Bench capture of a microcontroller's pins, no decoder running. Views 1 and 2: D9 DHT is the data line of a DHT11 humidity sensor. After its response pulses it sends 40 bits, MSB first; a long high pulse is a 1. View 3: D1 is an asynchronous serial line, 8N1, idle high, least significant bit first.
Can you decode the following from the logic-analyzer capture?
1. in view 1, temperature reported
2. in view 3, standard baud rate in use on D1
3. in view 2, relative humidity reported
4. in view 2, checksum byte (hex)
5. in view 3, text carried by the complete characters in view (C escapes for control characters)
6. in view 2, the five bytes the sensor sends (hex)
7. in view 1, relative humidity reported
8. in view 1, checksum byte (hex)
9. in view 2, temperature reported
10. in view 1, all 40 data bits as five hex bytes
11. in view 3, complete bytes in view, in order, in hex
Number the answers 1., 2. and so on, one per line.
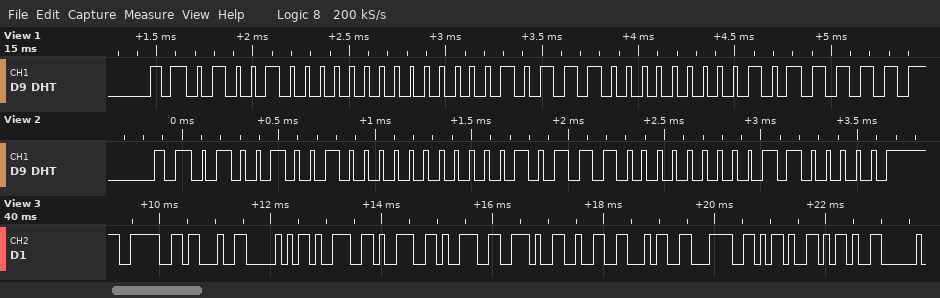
1. 23.0 °C
2. 9600 baud
3. 73 %
4. 0x60
5. ">#P999.24<--"
6. 49 00 17 00 60
7. 72 %
8. 0x5F
9. 23.0 °C
10. 48 00 17 00 5F
11. 3E 23 50 39 39 39 2E 32 34 3C 2D 2D
